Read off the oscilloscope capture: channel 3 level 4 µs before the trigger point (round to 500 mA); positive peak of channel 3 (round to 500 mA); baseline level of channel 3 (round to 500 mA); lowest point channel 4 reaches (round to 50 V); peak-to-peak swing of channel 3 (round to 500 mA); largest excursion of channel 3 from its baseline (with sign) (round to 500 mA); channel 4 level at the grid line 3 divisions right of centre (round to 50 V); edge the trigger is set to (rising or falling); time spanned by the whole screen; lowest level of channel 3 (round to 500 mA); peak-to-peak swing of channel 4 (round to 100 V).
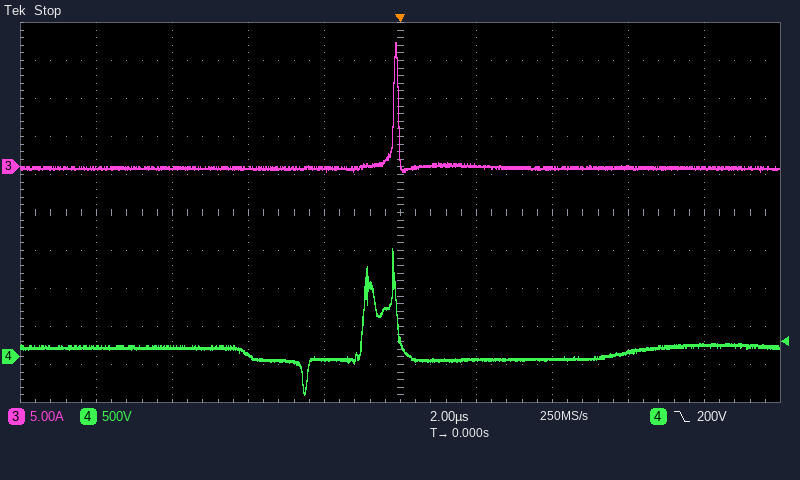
0.0 A
16.5 A
0.0 A
-500 V
17.0 A
+16.5 A
50 V
falling
20 µs
-500 mA
1.90 kV
